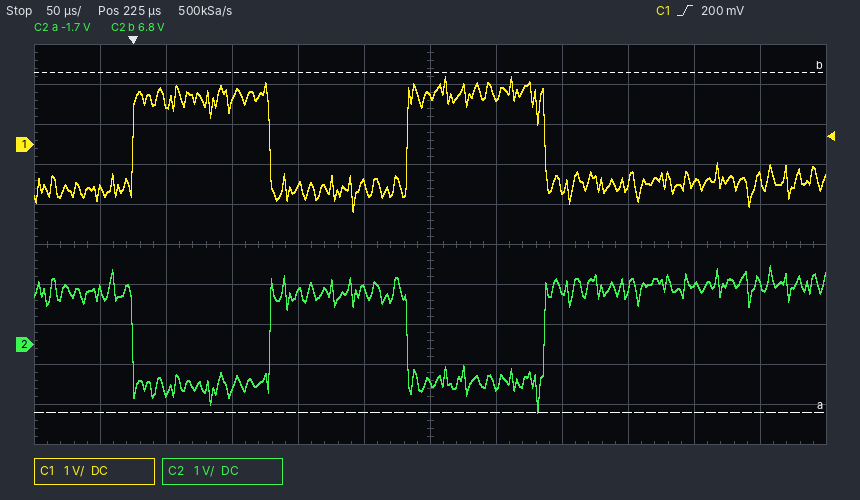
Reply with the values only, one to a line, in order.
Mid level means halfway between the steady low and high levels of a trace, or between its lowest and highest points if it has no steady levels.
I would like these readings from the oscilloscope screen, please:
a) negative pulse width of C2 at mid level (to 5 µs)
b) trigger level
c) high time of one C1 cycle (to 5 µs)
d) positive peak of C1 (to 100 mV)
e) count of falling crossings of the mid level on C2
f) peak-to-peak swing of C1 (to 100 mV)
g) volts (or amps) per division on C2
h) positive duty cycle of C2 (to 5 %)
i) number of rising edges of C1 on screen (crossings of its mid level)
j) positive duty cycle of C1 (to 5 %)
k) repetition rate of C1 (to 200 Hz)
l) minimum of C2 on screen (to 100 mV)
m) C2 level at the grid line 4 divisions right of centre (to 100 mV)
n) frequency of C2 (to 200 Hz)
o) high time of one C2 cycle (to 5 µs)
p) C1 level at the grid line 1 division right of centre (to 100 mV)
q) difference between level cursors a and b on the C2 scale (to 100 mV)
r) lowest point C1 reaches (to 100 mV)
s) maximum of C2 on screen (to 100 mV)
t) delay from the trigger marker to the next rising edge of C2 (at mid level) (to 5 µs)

105 µs
200 mV
105 µs
1.7 V
2
3.4 V
1 V
50 %
2
50 %
4.8 kHz
-1.7 V
1.5 V
4.8 kHz
105 µs
1.2 V
8.5 V
-1.7 V
2.0 V
105 µs
